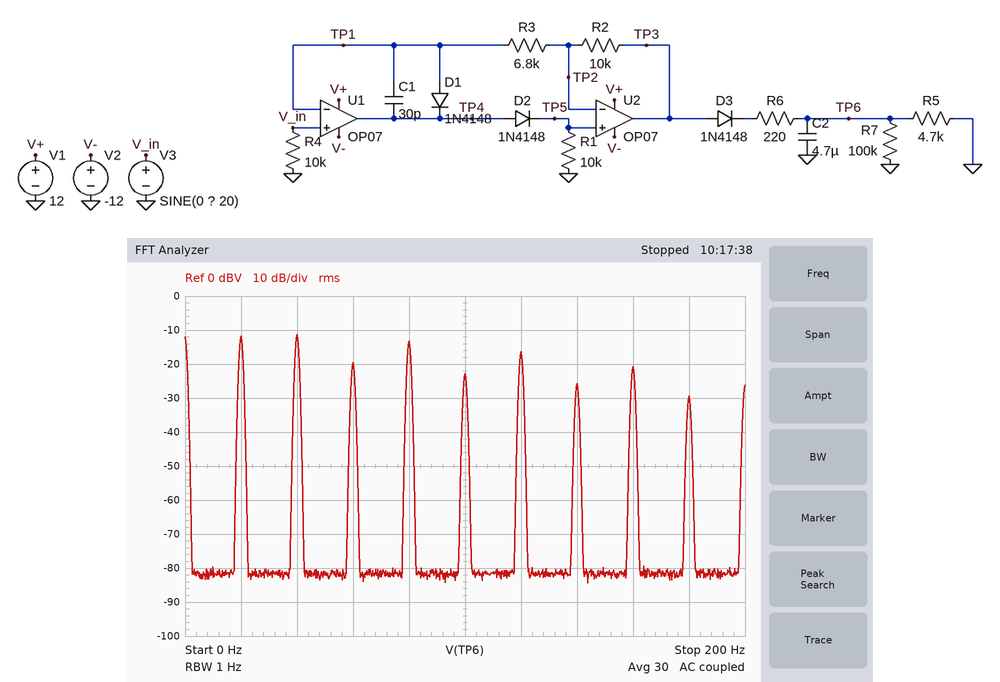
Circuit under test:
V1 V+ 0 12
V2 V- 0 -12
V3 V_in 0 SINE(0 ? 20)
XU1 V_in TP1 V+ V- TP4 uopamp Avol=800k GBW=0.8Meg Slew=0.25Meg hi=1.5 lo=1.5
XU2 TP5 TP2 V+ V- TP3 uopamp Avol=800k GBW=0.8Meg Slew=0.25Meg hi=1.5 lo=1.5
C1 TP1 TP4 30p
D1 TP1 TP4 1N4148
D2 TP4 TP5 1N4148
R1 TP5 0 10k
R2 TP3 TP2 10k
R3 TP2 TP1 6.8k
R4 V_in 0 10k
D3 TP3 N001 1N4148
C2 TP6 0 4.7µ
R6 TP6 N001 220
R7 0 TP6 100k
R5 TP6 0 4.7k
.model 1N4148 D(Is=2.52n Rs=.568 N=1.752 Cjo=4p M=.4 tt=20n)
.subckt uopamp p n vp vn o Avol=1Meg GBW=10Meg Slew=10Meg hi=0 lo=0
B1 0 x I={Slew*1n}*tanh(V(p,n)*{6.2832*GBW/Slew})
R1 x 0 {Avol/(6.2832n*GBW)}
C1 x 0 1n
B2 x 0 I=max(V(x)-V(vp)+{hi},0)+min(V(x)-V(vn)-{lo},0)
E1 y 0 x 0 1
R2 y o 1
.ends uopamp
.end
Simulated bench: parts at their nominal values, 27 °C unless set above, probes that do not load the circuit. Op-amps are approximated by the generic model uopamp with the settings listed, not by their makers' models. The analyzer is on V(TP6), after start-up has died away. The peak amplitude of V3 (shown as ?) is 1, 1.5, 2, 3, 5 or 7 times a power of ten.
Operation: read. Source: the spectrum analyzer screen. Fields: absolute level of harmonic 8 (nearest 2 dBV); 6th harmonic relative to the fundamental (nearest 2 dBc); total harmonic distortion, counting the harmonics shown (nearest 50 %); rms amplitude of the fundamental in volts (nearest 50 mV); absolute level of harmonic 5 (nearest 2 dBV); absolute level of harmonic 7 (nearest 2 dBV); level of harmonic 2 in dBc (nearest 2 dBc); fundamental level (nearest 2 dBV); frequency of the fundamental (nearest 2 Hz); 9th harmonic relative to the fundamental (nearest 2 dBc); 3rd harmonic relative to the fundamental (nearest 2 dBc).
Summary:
-20 dBV
-4 dBc
150 %
250 mV
-22 dBV
-26 dBV
0 dBc
-12 dBV
20 Hz
-18 dBc
-8 dBc
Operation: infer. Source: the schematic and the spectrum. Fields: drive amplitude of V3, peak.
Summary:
30 V
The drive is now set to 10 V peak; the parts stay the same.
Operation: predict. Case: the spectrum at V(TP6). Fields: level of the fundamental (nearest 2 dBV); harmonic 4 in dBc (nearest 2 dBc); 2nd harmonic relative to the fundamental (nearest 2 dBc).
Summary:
-4 dBV
-8 dBc
6 dBc
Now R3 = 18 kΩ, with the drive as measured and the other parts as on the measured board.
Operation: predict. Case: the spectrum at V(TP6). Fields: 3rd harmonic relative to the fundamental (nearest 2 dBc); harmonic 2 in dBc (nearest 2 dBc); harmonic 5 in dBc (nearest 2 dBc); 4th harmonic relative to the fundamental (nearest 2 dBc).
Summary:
-12 dBc
-18 dBc
-20 dBc
-16 dBc
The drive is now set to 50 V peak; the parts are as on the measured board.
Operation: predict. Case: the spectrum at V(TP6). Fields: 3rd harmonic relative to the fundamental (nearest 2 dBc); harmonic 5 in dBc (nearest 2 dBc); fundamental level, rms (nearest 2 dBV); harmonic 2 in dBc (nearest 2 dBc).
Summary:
-10 dBc
-14 dBc
-12 dBV
-6 dBc
